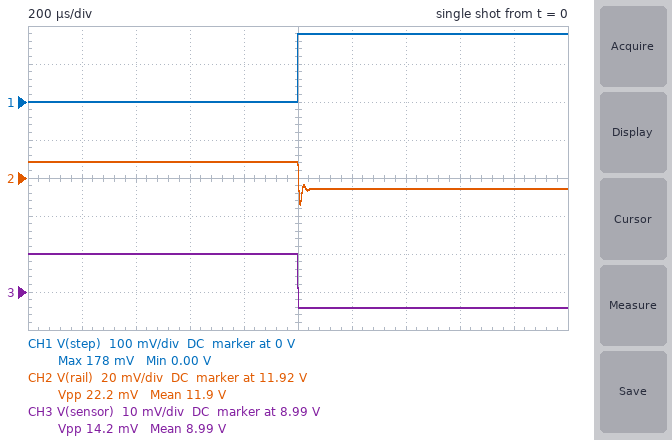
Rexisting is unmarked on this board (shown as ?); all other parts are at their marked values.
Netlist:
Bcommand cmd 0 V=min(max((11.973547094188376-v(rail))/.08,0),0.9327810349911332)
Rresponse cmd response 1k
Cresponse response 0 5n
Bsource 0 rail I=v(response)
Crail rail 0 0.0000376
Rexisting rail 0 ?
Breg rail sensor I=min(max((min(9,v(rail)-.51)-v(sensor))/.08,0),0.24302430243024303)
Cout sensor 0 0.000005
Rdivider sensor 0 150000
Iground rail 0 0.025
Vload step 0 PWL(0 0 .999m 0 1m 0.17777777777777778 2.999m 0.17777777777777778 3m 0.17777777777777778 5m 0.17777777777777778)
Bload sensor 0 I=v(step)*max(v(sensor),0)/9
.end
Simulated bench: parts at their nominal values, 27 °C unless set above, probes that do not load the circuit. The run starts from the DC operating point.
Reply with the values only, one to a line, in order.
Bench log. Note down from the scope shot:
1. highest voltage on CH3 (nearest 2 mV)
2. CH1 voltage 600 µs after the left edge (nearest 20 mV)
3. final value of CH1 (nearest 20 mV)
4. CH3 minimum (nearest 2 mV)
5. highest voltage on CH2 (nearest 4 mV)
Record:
9.000 V
0 V
180 mV
8.986 V
11.928 V
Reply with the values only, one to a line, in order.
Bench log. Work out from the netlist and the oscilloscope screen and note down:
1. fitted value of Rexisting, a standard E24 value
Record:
22 Ω
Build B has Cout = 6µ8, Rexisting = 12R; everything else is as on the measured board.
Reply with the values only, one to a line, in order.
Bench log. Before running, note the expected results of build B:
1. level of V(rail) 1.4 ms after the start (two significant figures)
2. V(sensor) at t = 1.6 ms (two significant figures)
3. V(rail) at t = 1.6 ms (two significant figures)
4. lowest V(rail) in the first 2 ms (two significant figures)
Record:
9.6 V
8.8 V
9.3 V
9.1 V
